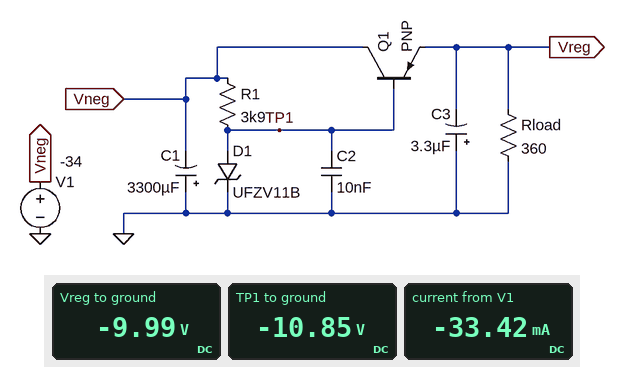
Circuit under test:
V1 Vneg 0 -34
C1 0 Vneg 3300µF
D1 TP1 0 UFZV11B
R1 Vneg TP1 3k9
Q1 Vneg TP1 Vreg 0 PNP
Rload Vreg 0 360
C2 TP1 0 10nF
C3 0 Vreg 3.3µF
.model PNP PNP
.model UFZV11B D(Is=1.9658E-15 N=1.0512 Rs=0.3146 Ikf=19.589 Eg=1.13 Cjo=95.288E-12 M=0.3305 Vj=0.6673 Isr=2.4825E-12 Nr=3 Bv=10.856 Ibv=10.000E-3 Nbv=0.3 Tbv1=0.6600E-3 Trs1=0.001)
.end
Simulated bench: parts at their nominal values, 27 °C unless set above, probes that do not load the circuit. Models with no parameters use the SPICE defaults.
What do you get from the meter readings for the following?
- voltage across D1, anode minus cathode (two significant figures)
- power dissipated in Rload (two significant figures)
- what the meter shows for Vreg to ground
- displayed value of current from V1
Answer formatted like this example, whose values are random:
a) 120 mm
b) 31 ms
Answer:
a) -11 V
b) 280 mW
c) -9.99 V
d) -33.42 mA
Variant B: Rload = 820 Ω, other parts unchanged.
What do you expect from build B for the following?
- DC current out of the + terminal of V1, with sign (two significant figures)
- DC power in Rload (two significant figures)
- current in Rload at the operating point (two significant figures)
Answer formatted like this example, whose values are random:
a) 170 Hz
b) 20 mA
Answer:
a) -18 mA
b) 120 mW
c) 12 mA
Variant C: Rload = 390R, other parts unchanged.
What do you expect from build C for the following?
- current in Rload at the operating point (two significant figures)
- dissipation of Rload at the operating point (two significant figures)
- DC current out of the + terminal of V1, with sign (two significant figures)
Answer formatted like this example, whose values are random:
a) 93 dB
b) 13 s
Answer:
a) 26 mA
b) 260 mW
c) -31 mA
